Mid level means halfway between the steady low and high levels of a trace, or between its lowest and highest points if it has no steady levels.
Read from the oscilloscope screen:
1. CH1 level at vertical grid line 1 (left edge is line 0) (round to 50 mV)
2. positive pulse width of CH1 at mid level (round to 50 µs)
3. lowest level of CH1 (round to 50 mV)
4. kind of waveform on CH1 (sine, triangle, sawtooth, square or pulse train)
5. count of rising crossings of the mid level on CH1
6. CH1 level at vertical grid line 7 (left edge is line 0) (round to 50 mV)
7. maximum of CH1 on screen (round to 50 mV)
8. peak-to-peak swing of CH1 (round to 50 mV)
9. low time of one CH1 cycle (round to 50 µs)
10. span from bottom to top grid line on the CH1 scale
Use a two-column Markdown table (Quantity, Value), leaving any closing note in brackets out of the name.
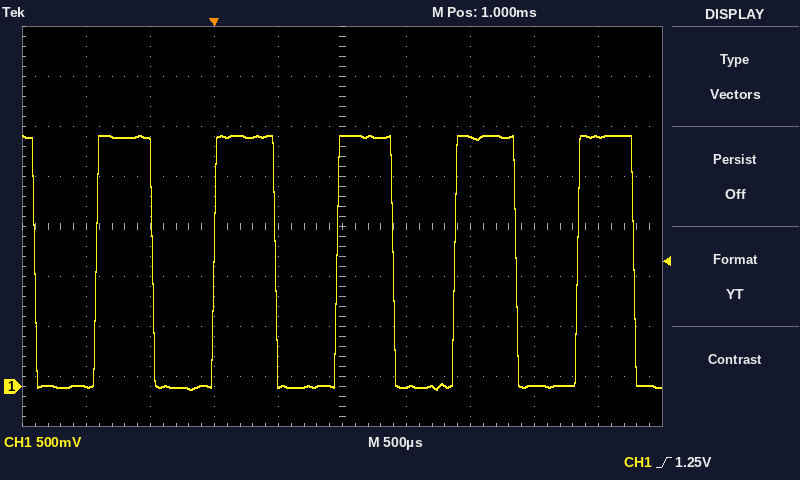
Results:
| Quantity | Value |
|---|---|
| CH1 level at vertical grid line 1 (left edge is line 0) | 0 mV |
| positive pulse width of CH1 at mid level | 450 µs |
| lowest level of CH1 | -50 mV |
| kind of waveform on CH1 | square |
| count of rising crossings of the mid level on CH1 | 5 |
| CH1 level at vertical grid line 7 (left edge is line 0) | 2.50 V |
| maximum of CH1 on screen | 2.50 V |
| peak-to-peak swing of CH1 | 2.55 V |
| low time of one CH1 cycle | 500 µs |
| span from bottom to top grid line on the CH1 scale | 4 V |
